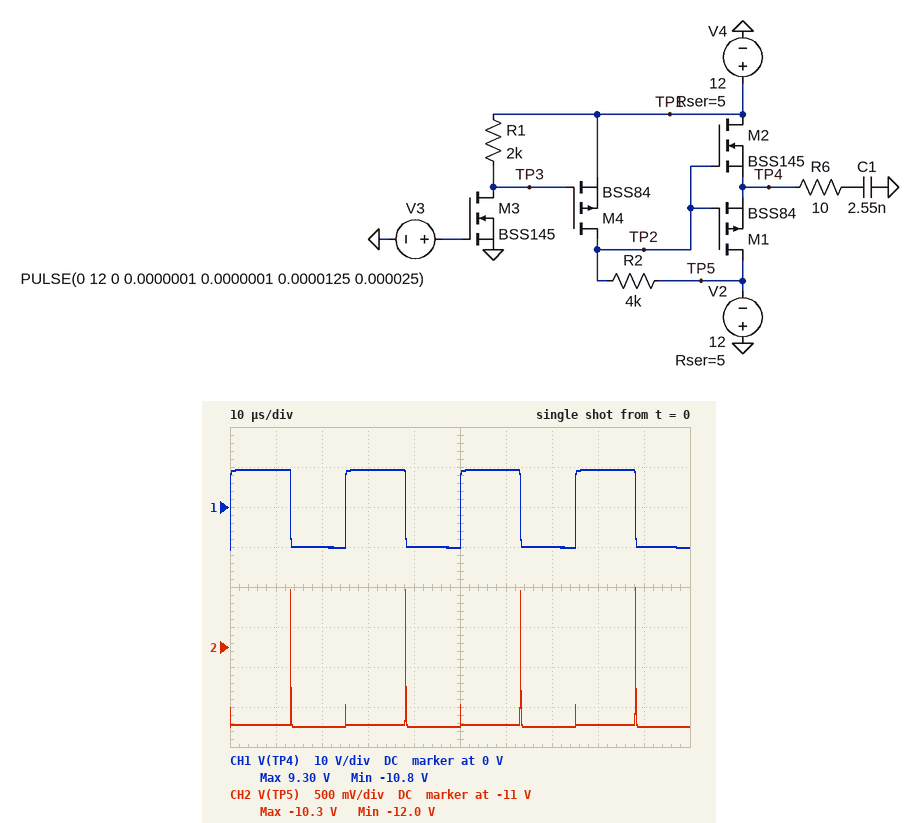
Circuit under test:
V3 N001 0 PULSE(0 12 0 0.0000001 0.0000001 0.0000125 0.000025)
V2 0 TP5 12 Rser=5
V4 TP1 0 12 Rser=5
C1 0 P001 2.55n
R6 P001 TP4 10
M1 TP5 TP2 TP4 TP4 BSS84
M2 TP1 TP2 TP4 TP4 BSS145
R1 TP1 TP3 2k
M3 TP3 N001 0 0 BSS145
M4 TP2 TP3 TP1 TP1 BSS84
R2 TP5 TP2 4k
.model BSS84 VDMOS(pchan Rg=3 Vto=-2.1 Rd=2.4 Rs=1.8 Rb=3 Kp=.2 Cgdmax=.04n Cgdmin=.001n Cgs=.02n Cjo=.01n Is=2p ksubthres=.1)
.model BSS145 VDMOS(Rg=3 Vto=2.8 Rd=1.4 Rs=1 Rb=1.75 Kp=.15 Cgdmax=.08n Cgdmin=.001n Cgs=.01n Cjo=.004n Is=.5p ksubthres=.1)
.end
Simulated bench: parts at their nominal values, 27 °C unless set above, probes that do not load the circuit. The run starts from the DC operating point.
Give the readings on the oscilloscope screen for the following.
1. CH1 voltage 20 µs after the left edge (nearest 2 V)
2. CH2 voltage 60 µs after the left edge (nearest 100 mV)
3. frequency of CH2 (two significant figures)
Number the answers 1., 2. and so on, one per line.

1. -10 V
2. -12.0 V
3. 40 kHz
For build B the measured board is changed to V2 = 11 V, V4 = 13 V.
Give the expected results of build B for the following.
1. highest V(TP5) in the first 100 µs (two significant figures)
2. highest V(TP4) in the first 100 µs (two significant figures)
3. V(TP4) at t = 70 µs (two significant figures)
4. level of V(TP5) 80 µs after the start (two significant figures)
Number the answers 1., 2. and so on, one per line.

1. -9.3 V
2. 10 V
3. -9.1 V
4. -11 V
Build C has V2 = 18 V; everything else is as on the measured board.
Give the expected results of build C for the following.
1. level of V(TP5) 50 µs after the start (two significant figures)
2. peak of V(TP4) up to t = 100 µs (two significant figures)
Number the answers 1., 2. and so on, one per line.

1. -18 V
2. 9.3 V
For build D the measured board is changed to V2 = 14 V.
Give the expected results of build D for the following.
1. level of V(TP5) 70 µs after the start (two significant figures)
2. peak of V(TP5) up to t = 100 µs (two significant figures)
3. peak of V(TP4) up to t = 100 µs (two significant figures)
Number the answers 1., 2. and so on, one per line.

1. -14 V
2. -12 V
3. 9.3 V
